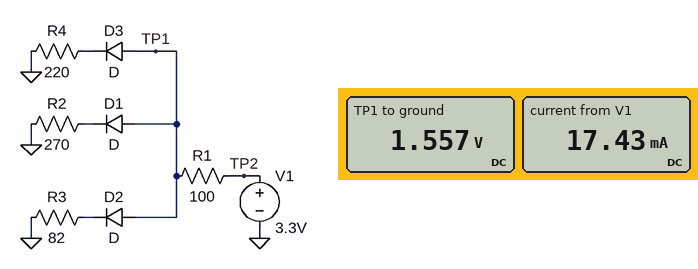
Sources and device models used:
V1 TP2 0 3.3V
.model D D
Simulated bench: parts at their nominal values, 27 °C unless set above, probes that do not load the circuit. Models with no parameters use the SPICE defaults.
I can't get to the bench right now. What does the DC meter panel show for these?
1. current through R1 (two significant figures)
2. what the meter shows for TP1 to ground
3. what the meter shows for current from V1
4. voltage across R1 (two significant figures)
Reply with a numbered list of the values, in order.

1. 17 mA
2. 1.557 V
3. 17.43 mA
4. 1.7 V
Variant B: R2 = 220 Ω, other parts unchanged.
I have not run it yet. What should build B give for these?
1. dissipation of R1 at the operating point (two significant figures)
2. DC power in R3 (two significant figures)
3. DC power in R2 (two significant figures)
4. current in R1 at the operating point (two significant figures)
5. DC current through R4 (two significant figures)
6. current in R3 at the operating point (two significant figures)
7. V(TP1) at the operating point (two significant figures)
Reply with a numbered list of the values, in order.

1. 31 mW
2. 8.2 mW
3. 3.2 mW
4. 18 mA
5. 3.8 mA
6. 10 mA
7. 1.5 V
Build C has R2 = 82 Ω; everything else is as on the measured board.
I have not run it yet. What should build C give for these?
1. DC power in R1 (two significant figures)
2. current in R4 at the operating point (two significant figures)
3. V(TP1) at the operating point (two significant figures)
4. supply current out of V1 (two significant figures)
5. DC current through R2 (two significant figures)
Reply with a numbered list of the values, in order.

1. 37 mW
2. 3.1 mA
3. 1.4 V
4. 19 mA
5. 8.1 mA
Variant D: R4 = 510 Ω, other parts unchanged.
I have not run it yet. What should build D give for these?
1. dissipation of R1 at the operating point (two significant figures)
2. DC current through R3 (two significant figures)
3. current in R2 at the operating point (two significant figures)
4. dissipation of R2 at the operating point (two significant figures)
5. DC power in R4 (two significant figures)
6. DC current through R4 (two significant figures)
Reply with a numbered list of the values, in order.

1. 28 mW
2. 11 mA
3. 3.5 mA
4. 3.3 mW
5. 1.8 mW
6. 1.9 mA
